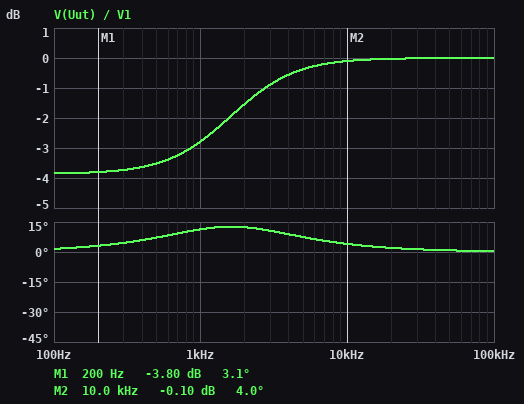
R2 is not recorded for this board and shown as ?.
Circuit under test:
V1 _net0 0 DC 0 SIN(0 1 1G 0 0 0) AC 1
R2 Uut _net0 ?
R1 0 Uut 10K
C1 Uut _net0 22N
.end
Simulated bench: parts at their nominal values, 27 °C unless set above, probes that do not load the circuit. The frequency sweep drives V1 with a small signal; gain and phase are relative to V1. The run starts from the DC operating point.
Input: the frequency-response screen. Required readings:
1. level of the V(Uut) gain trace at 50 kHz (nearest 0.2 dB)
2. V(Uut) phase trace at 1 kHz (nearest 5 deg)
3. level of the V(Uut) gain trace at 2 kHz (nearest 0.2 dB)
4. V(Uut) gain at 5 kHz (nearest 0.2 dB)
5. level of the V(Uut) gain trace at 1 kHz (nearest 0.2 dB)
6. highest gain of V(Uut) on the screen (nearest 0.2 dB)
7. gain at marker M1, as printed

0 dB
10 deg
-1.6 dB
-0.4 dB
-2.8 dB
0 dB
-3.80 dB
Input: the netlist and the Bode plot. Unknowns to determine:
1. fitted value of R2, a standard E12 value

5.6 kΩ
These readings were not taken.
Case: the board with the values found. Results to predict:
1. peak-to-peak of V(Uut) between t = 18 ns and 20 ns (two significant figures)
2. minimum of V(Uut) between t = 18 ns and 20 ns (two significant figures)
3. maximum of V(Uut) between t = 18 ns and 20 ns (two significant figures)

2.0 V
-1.0 V
1.0 V
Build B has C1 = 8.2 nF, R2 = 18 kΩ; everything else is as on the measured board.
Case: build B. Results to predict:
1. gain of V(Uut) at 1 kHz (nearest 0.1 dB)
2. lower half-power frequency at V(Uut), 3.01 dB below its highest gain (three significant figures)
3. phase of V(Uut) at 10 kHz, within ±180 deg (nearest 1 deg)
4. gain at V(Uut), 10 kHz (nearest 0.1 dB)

-6.7 dB
2.61 kHz
11 deg
-0.3 dB
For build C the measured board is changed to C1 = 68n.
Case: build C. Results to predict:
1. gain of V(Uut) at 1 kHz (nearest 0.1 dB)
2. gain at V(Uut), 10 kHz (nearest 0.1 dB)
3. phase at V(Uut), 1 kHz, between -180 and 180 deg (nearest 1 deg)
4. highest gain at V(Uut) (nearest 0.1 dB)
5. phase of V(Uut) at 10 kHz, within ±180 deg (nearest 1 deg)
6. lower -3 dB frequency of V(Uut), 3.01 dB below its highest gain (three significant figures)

-0.8 dB
0 dB
10 deg
0 dB
1 deg
275 Hz
